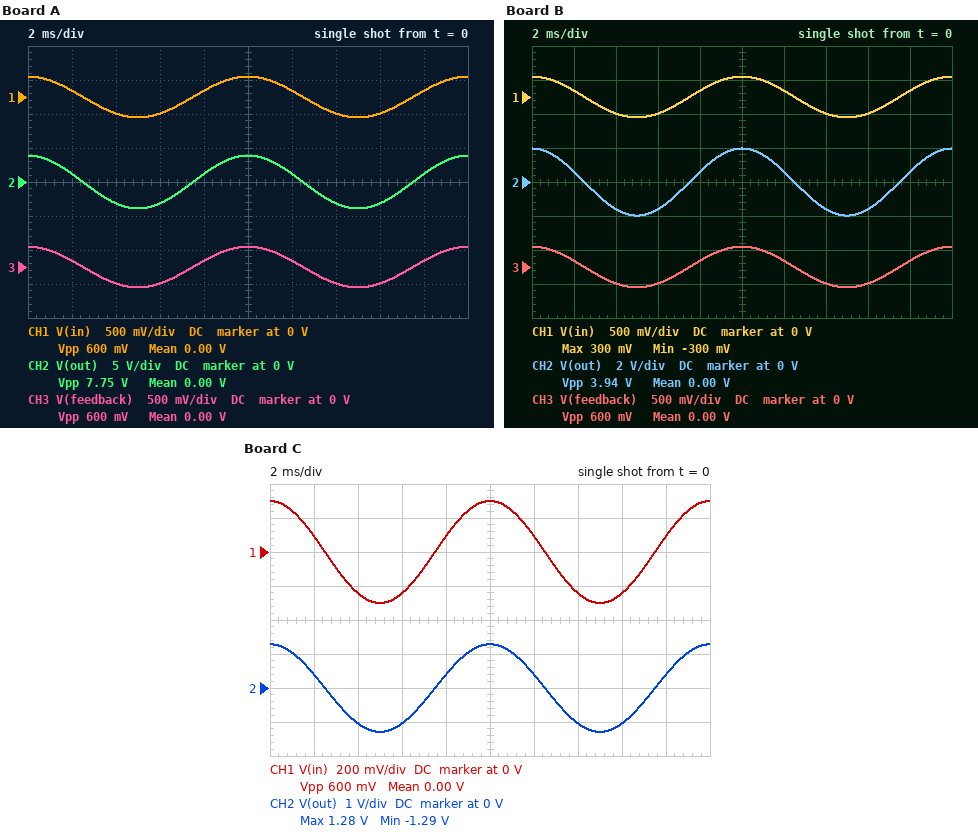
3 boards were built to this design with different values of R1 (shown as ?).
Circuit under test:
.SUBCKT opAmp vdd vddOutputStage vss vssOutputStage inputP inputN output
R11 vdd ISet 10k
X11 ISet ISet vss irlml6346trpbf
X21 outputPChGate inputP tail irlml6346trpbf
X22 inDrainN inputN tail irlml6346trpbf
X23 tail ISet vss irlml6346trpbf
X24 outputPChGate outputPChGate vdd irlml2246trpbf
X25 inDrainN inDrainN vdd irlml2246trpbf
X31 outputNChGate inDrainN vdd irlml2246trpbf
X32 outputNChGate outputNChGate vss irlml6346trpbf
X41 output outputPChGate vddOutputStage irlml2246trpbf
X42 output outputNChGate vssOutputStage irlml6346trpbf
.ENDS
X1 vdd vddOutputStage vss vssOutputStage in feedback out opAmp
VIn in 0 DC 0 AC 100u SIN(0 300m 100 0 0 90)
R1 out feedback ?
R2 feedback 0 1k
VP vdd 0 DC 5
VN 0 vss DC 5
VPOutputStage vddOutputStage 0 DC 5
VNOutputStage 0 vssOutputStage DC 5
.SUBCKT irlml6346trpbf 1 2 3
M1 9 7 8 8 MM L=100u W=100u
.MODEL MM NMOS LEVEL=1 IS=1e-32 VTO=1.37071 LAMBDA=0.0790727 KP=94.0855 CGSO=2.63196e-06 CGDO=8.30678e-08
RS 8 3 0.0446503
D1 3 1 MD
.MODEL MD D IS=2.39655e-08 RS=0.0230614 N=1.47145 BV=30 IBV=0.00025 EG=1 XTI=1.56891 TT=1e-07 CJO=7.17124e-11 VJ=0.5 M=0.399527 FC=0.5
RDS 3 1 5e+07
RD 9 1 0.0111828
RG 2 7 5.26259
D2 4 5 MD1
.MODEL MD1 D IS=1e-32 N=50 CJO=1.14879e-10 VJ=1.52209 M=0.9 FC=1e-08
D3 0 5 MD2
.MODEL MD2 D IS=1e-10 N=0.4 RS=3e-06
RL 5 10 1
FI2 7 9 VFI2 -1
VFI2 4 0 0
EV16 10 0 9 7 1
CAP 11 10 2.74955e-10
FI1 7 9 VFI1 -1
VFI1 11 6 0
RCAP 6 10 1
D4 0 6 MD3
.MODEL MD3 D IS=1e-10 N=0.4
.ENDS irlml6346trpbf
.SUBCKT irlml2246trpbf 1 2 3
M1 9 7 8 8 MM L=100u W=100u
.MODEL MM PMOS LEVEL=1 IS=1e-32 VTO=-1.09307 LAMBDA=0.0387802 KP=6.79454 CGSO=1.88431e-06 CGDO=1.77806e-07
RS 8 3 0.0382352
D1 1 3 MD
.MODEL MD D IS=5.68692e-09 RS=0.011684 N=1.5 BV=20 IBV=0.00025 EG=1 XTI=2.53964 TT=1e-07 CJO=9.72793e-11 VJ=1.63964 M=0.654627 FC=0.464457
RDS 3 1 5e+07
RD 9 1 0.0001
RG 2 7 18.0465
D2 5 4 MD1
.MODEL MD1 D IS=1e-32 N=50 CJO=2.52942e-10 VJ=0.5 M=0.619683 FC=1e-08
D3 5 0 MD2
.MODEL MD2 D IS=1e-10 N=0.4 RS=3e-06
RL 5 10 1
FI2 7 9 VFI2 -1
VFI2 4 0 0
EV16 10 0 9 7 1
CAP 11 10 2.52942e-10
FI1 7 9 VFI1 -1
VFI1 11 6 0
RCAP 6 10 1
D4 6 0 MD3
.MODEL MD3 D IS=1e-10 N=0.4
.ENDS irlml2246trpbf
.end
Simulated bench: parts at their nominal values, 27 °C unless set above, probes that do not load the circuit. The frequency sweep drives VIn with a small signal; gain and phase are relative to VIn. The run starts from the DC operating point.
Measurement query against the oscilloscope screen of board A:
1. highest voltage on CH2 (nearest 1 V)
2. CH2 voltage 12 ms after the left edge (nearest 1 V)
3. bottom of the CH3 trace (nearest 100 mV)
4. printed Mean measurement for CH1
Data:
4 V
1 V
-300 mV
0.00 V
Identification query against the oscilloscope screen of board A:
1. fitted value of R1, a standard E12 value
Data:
12 kΩ
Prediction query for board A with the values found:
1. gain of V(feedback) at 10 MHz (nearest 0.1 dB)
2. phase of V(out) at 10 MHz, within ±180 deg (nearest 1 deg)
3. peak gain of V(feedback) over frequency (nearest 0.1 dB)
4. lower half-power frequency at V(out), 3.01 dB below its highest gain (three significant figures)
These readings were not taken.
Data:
-1.7 dB
-116 deg
2.4 dB
2.17 MHz
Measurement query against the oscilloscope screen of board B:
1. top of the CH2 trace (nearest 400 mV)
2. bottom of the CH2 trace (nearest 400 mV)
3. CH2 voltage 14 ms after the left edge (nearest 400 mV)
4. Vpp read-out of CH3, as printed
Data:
2.0 V
-2.0 V
-1.6 V
600 mV
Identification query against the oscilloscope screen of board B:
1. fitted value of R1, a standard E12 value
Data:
5.6 kΩ
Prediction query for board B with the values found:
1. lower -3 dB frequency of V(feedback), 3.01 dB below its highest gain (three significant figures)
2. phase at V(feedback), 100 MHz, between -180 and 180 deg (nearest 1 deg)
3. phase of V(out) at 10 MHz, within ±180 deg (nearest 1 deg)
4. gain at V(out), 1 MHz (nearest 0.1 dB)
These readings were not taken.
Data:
3.22 MHz
-33 deg
-119 deg
17.3 dB
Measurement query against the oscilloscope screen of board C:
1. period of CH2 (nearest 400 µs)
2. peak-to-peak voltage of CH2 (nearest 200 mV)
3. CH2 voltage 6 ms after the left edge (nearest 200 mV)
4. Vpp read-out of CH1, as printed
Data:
10.0 ms
2.6 V
-1.0 V
600 mV
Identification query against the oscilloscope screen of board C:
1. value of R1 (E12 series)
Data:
3.3 kΩ
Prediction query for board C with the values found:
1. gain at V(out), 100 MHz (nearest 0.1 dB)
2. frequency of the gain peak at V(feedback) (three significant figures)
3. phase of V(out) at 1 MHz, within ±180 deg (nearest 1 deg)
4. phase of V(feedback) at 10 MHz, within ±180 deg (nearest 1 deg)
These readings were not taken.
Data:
-17.3 dB
4.55 MHz
10 deg
0 deg
